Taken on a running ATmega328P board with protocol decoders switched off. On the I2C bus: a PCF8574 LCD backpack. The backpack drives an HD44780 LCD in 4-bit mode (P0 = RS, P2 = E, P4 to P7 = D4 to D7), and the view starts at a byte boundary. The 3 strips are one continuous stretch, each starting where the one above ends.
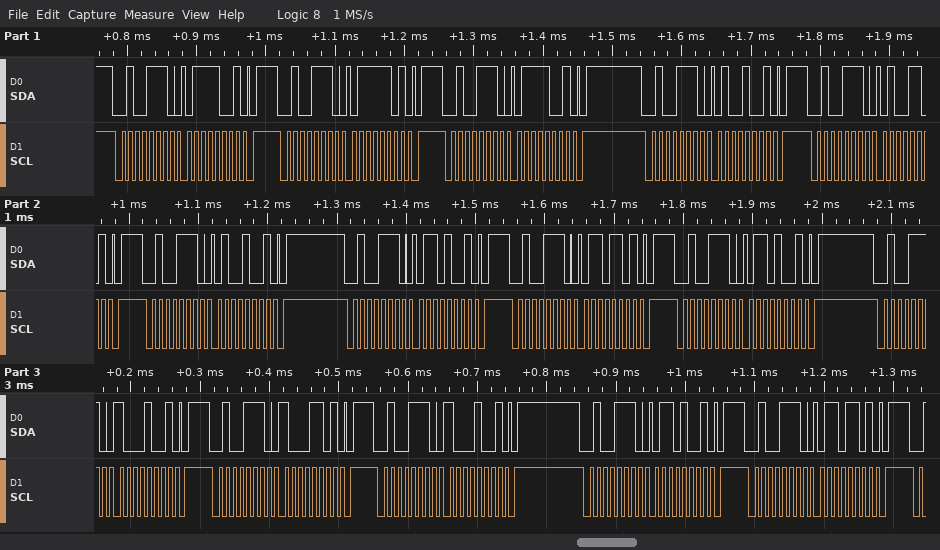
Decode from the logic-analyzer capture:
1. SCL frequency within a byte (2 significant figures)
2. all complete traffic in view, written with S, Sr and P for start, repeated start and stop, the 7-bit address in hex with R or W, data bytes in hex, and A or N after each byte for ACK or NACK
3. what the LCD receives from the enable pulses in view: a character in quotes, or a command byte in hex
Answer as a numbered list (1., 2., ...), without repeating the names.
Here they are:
1. 100 kHz
2. S 27W A 79 A P S 27W A 7D A P S 27W A 79 A P S 27W A 49 A P S 27W A 4D A P S 27W A 49 A P S 27W A 69 A P S 27W A 6D A P S 27W A 69 A P S 27W A 89 A P S 27W A 8D A P S 27W A 89 A P S 27W A 69 A P S 27W A 6D A P
3. 't' 'h'
